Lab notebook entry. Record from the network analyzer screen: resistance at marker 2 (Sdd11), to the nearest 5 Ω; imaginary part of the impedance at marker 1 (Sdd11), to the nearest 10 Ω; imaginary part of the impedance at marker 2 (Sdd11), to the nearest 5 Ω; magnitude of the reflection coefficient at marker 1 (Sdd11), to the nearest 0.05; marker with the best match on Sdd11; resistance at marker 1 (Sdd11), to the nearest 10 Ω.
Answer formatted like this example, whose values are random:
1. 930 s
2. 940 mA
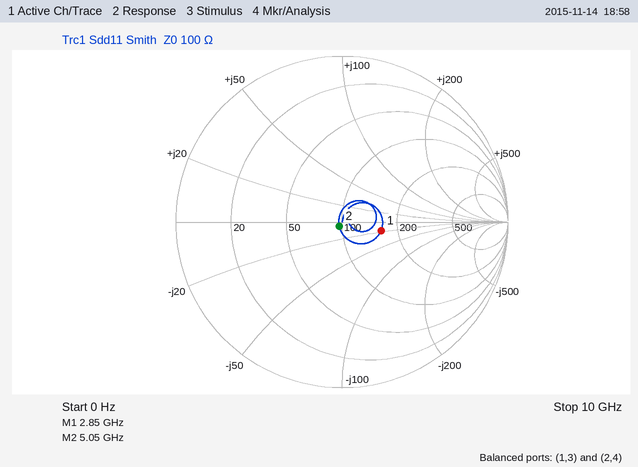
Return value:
1. 95 Ω
2. -20 Ω
3. -5 Ω
4. 0.25
5. marker 2
6. 160 Ω
